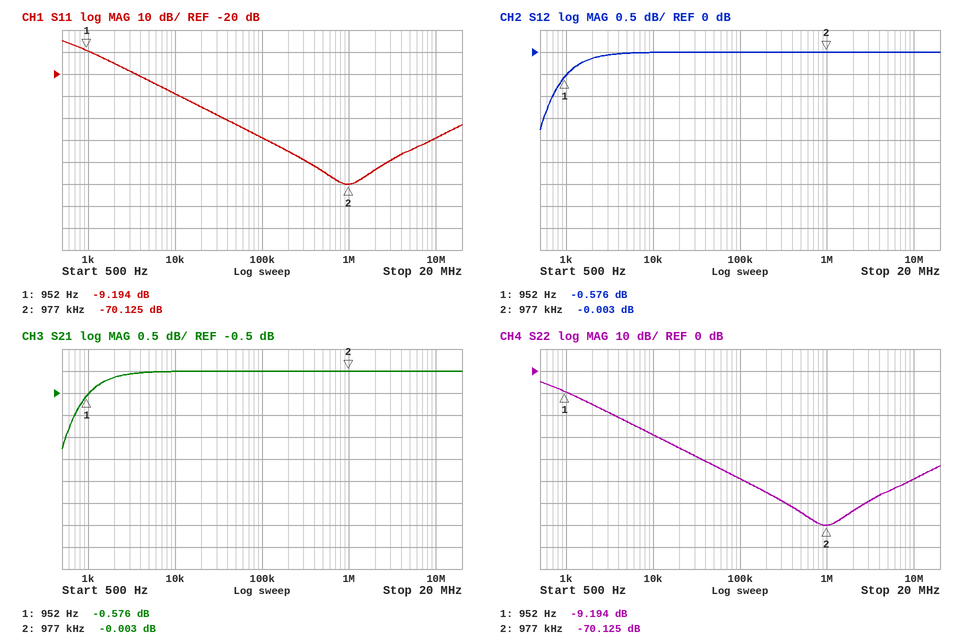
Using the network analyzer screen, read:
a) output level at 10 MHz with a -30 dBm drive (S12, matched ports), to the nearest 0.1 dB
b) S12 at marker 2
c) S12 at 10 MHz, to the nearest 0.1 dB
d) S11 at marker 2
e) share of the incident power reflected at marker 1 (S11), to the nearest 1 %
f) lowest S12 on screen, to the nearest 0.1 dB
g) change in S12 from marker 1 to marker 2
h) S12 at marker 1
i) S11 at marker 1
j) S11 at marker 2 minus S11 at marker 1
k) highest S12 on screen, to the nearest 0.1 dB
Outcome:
-30.0 dBm
-0.003 dB
0.0 dB
-70.125 dB
12 %
-1.8 dB
0.573 dB
-0.576 dB
-9.194 dB
-60.931 dB
0.0 dB
